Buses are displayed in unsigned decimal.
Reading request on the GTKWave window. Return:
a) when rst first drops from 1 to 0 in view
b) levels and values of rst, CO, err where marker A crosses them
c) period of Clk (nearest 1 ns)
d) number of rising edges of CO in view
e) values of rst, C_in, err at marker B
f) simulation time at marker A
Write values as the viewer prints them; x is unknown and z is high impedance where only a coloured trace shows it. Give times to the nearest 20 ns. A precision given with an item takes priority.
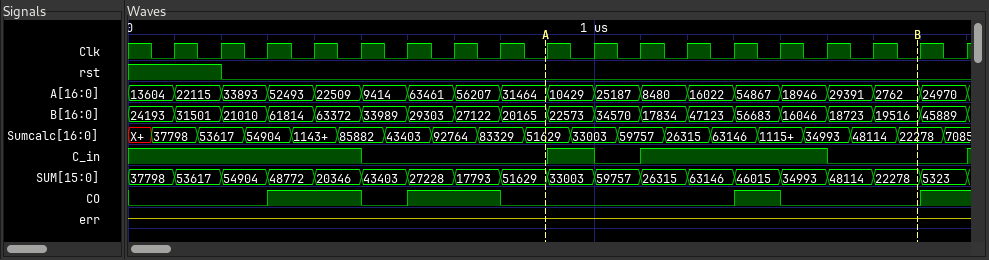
200 ns
rst=0, CO=0, err=z
100 ns
4
rst=0, C_in=0, err=z
900 ns
